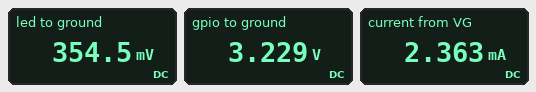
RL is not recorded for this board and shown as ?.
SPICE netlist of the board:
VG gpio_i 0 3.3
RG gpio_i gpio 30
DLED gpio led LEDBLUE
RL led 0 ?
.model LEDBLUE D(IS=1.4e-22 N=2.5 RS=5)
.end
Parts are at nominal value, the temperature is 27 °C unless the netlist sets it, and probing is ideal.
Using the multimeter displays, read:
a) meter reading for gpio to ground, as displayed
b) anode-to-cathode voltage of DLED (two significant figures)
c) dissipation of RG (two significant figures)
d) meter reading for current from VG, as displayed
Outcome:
3.229 V
2.9 V
170 µW
2.363 mA
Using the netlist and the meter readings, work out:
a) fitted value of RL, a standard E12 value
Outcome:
150 Ω
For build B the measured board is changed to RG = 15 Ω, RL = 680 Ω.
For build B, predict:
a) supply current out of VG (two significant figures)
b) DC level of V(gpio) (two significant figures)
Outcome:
730 µA
3.3 V
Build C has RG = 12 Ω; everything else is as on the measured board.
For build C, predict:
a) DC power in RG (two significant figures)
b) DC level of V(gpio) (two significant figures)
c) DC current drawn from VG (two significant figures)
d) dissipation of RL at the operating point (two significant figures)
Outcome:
80 µW
3.3 V
2.6 mA
1.0 mW
